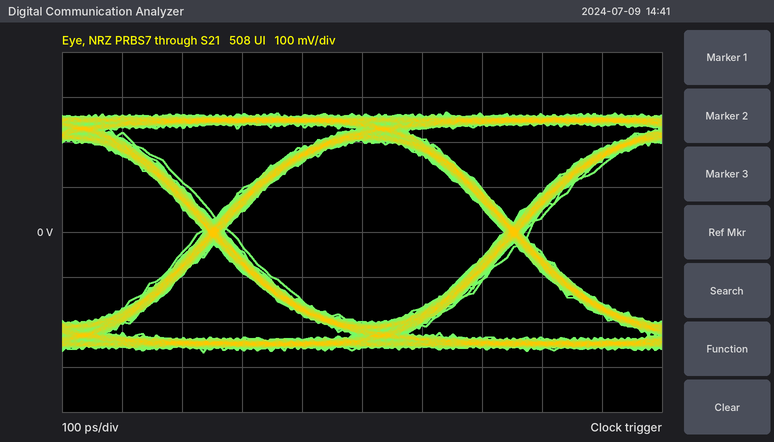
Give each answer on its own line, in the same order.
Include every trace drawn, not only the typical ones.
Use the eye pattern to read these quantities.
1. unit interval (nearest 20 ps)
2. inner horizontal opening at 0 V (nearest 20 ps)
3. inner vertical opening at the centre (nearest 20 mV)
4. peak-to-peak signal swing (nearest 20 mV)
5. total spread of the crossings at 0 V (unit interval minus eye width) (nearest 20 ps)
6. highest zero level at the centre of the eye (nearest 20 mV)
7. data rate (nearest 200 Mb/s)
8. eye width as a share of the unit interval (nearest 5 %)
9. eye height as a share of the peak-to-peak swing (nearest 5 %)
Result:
500 ps
460 ps
400 mV
540 mV
40 ps
-200 mV
2.0 Gb/s
90 %
75 %
